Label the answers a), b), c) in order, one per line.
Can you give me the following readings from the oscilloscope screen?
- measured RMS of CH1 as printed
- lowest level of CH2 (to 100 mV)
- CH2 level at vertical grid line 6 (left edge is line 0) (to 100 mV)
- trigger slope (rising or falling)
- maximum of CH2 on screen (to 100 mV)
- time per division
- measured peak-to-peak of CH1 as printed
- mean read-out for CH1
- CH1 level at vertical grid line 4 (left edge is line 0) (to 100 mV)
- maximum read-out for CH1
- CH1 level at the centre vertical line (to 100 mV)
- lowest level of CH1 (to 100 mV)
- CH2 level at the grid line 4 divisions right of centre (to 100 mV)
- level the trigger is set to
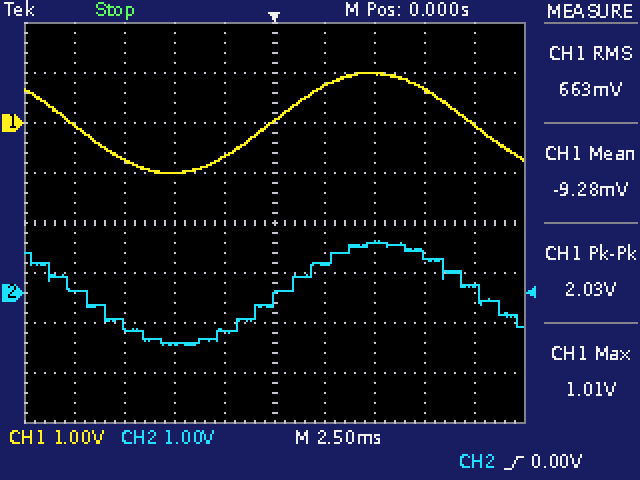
a) 663 mV
b) -1.0 V
c) 600 mV
d) rising
e) 1.0 V
f) 2.5 ms
g) 2.03 V
h) -9.28 mV
i) -700 mV
j) 1.01 V
k) 0.0 V
l) -1.0 V
m) 100 mV
n) 0.00 V
